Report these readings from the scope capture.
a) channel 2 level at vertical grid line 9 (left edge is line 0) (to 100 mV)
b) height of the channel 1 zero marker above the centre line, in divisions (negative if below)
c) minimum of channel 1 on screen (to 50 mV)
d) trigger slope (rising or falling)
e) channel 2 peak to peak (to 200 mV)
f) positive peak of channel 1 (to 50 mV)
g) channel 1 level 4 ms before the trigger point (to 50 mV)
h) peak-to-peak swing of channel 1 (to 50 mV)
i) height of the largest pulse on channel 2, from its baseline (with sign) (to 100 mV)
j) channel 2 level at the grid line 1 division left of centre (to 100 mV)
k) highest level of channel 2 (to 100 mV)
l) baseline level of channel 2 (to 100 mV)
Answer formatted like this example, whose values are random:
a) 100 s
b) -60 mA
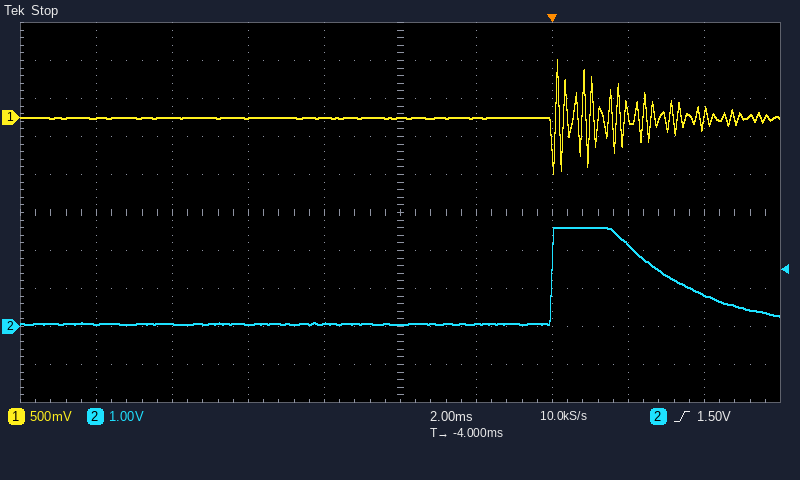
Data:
a) 800 mV
b) +2.5 div
c) -750 mV
d) rising
e) 2.6 V
f) 750 mV
g) 0 mV
h) 1.50 V
i) +2.5 V
j) 100 mV
k) 2.6 V
l) 100 mV
